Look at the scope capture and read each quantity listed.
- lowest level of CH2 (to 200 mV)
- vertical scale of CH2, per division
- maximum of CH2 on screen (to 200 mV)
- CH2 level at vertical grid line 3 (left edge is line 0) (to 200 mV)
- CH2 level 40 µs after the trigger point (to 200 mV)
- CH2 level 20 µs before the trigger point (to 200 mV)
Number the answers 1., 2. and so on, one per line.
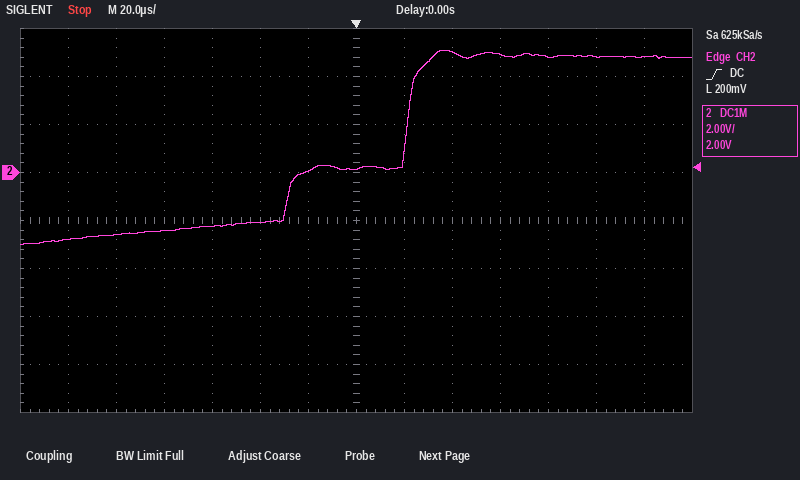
1. -3.0 V
2. 2 V
3. 5.0 V
4. -2.4 V
5. 5.0 V
6. 0.0 V
